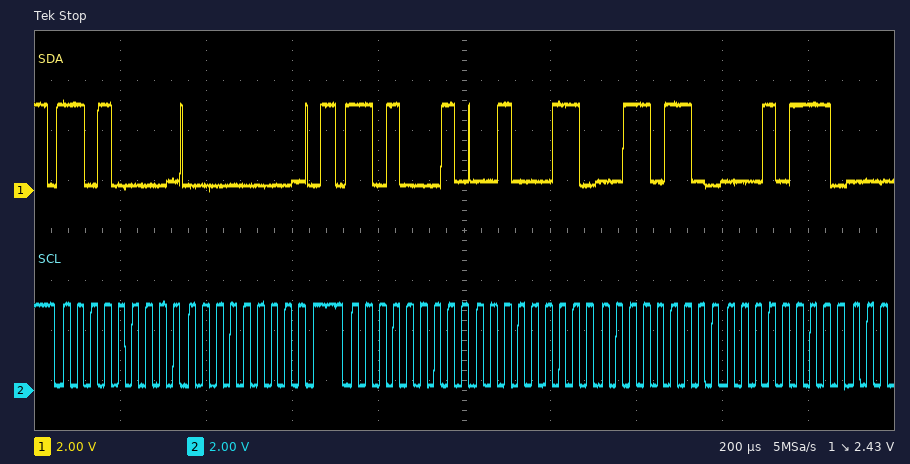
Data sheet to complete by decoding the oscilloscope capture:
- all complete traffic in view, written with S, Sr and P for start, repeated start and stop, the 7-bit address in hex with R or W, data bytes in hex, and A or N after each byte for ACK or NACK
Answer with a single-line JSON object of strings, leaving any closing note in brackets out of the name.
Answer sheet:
{"all complete traffic in view, written with S, Sr and P for start, repeated start and stop, the 7-bit address in hex with R or W, data bytes in hex, and A or N after each byte for ACK or NACK": "S 68W A 00 A P S 68R A 23 A 36 A 17 A"}
